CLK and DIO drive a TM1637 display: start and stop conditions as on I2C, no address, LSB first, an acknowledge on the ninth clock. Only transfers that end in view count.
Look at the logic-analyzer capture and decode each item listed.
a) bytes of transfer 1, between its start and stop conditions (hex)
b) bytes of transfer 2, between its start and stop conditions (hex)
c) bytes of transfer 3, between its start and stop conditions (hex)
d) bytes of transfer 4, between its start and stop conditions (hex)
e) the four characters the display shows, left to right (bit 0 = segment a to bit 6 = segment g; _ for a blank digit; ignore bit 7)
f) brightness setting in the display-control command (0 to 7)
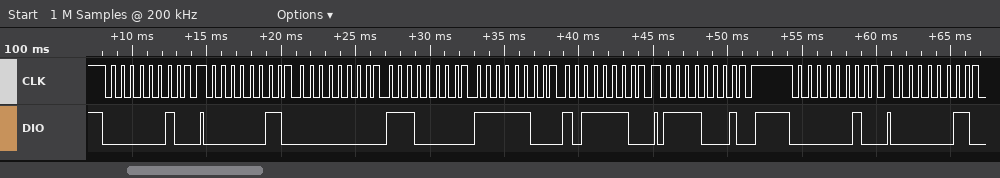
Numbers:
40
C0 00 07 3F 7D
8F
40
_706
7
